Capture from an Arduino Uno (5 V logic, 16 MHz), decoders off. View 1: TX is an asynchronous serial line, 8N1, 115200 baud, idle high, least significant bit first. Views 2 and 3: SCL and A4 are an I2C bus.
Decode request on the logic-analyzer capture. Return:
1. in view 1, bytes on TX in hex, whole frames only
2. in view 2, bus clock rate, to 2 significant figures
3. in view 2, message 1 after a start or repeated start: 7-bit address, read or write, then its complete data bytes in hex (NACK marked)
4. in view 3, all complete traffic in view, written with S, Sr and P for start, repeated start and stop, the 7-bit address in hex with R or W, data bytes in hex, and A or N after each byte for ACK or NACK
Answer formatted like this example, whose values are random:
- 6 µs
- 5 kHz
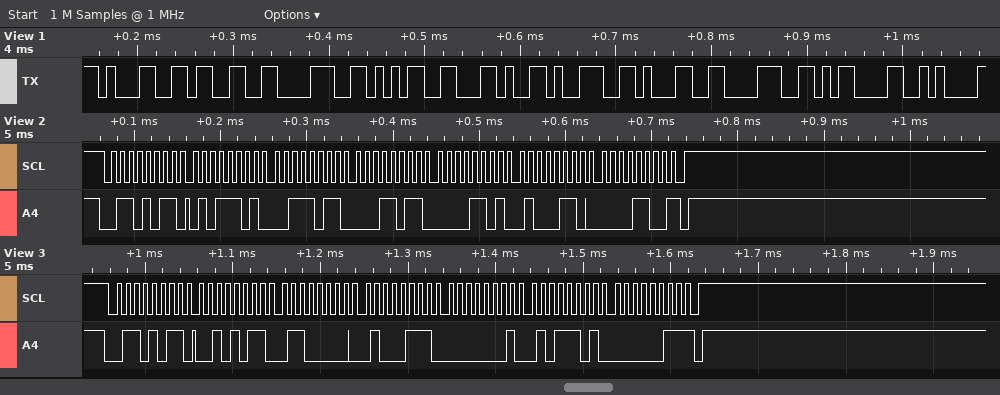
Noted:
- 31 33 38 35 2C 39 31 38 0D 0A
- 100 kHz
- 0x35 read: 5D 3B 1B 0D 46 0C NACK
- S 35R A 2B A 60 A 47 A 01 A 5D A 03 N P
